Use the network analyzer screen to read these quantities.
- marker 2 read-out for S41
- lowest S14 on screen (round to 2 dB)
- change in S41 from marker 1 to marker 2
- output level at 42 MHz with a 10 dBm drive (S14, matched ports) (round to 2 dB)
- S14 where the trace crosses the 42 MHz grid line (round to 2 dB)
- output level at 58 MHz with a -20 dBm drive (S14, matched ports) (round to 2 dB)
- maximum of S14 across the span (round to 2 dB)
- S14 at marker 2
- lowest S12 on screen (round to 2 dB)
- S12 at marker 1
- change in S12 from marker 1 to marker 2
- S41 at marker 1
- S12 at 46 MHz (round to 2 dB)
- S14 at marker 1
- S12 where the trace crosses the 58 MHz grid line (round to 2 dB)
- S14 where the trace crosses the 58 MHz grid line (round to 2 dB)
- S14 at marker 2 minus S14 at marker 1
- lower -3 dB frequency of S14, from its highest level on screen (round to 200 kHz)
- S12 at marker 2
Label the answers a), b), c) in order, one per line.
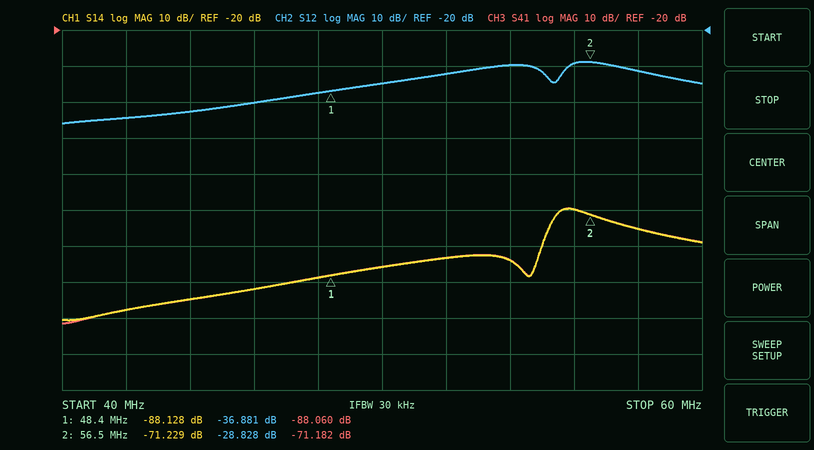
a) -71.182 dB
b) -100 dB
c) 16.878 dB
d) -88 dBm
e) -98 dB
f) -96 dBm
g) -70 dB
h) -71.229 dB
i) -46 dB
j) -36.881 dB
k) 8.053 dB
l) -88.060 dB
m) -40 dB
n) -88.128 dB
o) -32 dB
p) -76 dB
q) 16.899 dB
r) 55.4 MHz
s) -28.828 dB
